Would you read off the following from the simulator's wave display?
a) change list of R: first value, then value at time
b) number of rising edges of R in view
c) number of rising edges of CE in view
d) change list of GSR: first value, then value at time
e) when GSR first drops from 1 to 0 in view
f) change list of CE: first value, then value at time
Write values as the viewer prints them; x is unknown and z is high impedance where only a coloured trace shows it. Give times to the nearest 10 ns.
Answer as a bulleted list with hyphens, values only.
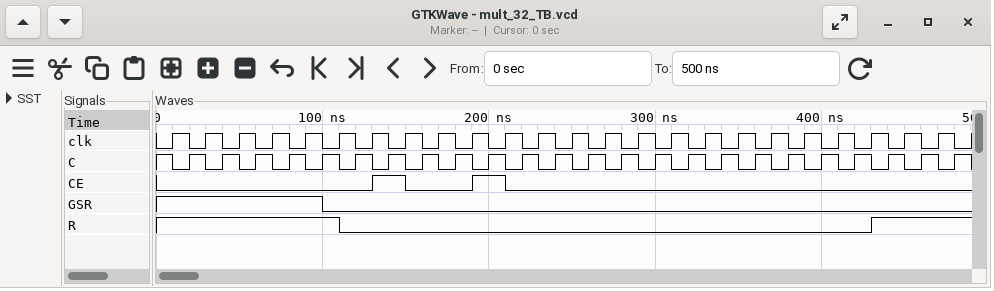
- 1, 0 at 110 ns, 1 at 430 ns
- 1
- 2
- 1, 0 at 100 ns
- 100 ns
- 0, 1 at 130 ns, 0 at 150 ns, 1 at 190 ns, 0 at 210 ns
